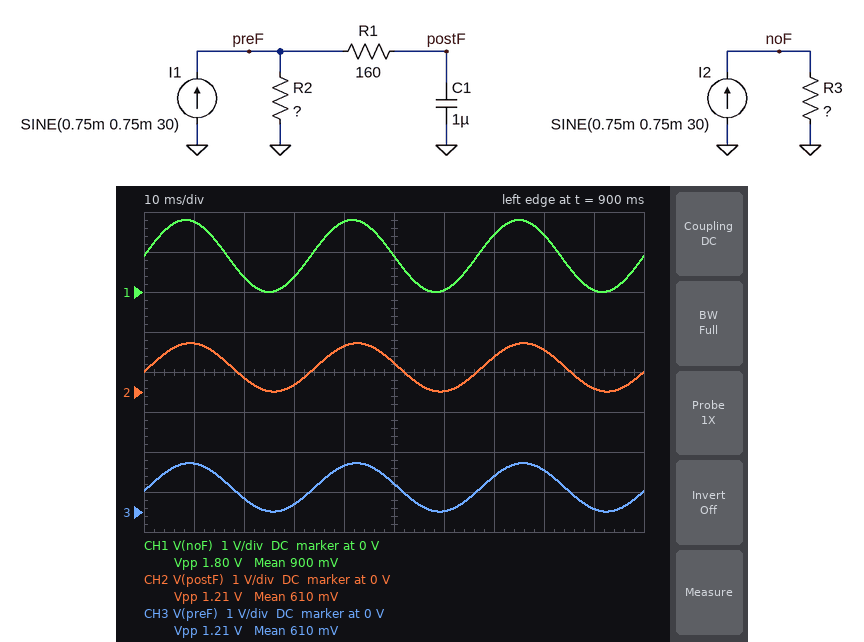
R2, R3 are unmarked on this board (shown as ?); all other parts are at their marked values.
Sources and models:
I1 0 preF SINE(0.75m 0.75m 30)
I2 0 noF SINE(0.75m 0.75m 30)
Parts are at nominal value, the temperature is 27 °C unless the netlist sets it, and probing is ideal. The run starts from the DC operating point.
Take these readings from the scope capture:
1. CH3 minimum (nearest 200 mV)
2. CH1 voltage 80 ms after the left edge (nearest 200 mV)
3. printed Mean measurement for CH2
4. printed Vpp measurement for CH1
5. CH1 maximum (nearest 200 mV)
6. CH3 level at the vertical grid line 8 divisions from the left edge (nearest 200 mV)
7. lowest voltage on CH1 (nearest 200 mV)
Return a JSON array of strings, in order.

["0 V", "1.4 V", "610 mV", "1.80 V", "1.8 V", "1.0 V", "0 V"]
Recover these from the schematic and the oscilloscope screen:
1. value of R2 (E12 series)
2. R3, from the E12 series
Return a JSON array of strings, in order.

["820 Ω", "1.2 kΩ"]
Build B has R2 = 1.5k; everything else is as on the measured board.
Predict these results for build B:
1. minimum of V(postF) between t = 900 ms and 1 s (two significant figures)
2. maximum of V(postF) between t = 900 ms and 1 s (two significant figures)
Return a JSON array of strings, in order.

["51 mV", "2.2 V"]
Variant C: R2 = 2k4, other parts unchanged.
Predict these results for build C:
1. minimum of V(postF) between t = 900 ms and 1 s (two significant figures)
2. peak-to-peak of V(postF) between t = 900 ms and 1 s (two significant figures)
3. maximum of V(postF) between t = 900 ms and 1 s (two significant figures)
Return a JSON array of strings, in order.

["180 mV", "3.2 V", "3.4 V"]
